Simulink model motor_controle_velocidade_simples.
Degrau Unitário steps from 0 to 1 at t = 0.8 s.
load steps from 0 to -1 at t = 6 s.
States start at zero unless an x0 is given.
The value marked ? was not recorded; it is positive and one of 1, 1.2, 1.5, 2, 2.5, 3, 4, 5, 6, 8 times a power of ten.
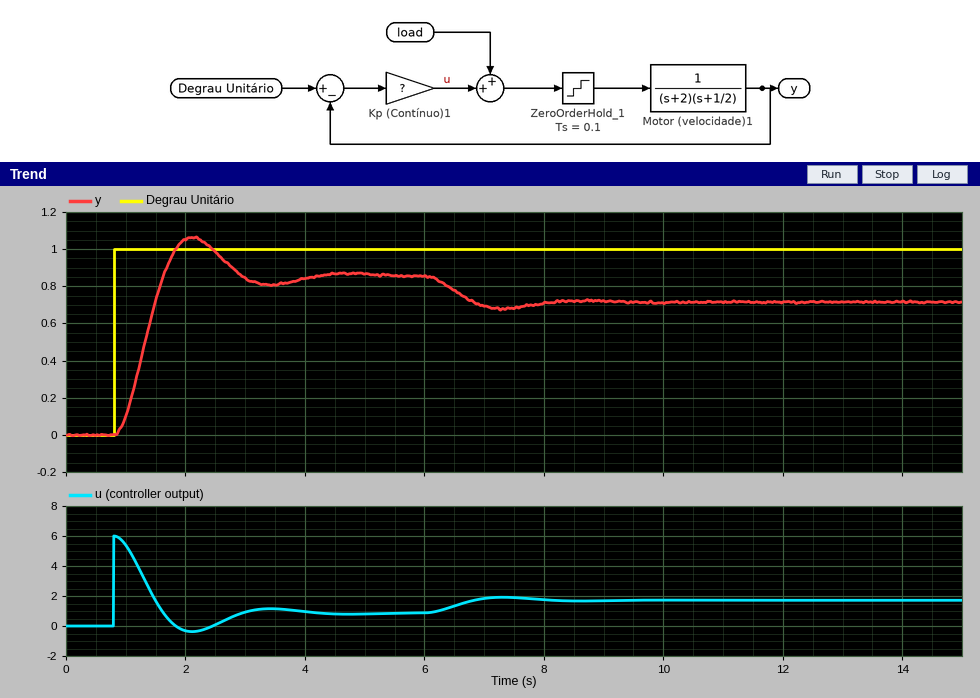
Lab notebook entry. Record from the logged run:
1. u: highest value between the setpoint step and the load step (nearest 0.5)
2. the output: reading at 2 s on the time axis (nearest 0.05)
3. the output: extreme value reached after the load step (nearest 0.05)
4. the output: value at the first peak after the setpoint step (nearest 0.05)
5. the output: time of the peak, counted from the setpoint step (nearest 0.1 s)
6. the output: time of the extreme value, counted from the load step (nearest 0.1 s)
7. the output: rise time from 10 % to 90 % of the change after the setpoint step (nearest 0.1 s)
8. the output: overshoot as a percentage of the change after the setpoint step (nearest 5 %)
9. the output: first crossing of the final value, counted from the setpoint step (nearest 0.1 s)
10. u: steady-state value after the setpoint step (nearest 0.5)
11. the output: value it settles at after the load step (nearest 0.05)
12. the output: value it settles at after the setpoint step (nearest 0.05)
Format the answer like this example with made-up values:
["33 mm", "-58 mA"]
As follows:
["6.0", "1.05", "0.70", "1.05", "1.3 s", "1.3 s", "0.6 s", "25 %", "0.8 s", "1.0", "0.70", "0.85"]
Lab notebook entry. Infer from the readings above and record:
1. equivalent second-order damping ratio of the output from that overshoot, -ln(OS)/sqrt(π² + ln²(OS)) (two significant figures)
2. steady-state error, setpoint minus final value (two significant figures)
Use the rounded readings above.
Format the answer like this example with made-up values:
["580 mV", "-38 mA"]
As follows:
["0.40", "0.15"]
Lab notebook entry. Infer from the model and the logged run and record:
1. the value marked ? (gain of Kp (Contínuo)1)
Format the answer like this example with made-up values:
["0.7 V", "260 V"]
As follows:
["6"]
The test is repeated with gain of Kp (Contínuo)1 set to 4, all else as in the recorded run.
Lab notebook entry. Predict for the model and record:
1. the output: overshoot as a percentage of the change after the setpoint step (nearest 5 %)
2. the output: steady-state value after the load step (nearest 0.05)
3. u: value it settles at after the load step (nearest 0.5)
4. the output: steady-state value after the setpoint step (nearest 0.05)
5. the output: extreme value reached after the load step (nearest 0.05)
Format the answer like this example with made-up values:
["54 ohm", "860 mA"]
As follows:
["15 %", "0.60", "1.5", "0.80", "0.55"]
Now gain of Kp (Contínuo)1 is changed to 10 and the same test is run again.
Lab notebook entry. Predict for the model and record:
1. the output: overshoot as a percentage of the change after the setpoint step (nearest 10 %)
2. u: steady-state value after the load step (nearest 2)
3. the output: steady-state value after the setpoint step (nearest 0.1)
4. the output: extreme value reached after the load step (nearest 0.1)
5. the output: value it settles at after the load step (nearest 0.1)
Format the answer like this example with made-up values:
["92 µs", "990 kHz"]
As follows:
["40 %", "2", "0.9", "0.8", "0.8"]
